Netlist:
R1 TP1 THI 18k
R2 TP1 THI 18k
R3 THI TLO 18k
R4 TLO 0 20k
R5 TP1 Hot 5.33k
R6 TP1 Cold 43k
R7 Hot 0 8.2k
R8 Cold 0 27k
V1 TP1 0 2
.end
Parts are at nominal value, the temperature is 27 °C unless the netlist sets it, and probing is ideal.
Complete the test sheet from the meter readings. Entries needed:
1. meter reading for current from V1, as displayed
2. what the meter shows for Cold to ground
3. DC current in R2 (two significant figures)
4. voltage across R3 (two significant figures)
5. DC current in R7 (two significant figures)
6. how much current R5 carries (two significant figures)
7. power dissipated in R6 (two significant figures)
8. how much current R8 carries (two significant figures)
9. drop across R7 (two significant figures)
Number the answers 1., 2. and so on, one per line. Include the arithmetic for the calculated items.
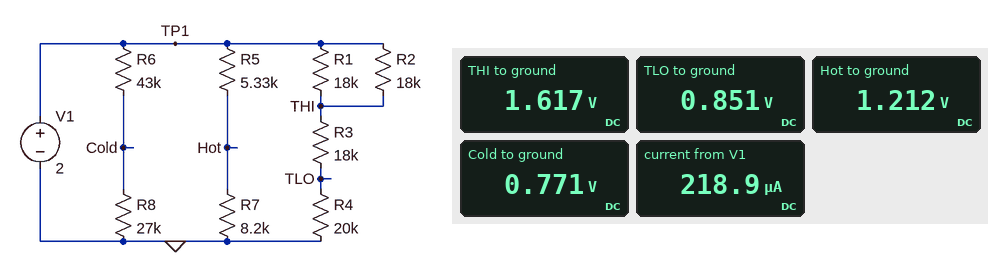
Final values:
1. 218.9 µA
2. 0.771 V
3. (2 V - 1.617 V) / 18 kΩ = 21 µA
4. 1.617 V - 851 mV = 770 mV
5. (1.212 V) / 8.2 kΩ = 150 µA
6. (2 V - 1.212 V) / 5.33 kΩ = 150 µA
7. (2 V - 771 mV)^2 / 43 kΩ = 35 µW
8. (771 mV) / 27 kΩ = 29 µA
9. 1.212 V = 1.2 V
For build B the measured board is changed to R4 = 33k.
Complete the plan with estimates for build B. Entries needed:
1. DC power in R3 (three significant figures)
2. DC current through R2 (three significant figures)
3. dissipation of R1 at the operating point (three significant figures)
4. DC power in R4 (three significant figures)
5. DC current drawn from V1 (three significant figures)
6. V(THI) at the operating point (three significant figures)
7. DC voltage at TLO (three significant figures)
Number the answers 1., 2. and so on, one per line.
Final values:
1. 20.0 µW
2. 16.7 µA
3. 5.00 µW
4. 36.7 µW
5. 210 µA
6. 1.70 V
7. 1.10 V
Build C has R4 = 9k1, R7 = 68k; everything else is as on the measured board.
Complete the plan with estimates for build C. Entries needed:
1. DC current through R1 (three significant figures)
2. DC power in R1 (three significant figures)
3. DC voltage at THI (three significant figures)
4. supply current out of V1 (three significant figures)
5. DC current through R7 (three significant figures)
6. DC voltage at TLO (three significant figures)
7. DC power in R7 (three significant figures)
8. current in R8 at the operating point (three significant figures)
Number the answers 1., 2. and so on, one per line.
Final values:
1. 27.7 µA
2. 13.8 µW
3. 1.50 V
4. 111 µA
5. 27.3 µA
6. 504 mV
7. 50.6 µW
8. 28.6 µA
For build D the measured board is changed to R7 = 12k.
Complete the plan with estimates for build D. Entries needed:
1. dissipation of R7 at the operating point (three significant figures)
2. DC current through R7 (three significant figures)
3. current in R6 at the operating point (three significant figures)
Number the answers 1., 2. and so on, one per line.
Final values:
1. 160 µW
2. 115 µA
3. 28.6 µA
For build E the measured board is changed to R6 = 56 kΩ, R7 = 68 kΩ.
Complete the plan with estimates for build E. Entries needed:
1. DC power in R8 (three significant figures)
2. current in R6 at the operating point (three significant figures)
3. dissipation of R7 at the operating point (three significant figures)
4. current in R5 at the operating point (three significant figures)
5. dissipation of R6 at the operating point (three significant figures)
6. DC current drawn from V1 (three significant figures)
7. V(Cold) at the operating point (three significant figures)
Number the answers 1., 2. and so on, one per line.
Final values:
1. 15.7 µW
2. 24.1 µA
3. 50.6 µW
4. 27.3 µA
5. 32.5 µW
6. 93.9 µA
7. 651 mV
